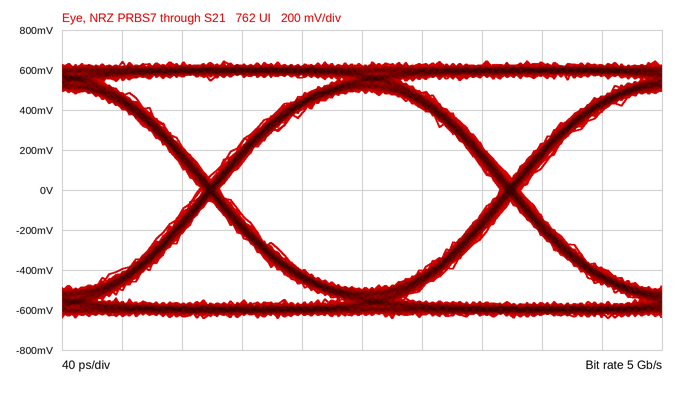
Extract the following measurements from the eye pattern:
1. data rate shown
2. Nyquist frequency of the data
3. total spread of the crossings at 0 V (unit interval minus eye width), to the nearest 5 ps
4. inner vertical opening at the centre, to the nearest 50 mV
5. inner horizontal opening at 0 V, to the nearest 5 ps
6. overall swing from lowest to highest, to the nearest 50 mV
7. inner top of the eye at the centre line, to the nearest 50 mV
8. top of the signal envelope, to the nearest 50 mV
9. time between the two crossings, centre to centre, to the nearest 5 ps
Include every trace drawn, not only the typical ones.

5 Gb/s
2.5 GHz
15 ps
1.00 V
185 ps
1.30 V
500 mV
650 mV
200 ps
